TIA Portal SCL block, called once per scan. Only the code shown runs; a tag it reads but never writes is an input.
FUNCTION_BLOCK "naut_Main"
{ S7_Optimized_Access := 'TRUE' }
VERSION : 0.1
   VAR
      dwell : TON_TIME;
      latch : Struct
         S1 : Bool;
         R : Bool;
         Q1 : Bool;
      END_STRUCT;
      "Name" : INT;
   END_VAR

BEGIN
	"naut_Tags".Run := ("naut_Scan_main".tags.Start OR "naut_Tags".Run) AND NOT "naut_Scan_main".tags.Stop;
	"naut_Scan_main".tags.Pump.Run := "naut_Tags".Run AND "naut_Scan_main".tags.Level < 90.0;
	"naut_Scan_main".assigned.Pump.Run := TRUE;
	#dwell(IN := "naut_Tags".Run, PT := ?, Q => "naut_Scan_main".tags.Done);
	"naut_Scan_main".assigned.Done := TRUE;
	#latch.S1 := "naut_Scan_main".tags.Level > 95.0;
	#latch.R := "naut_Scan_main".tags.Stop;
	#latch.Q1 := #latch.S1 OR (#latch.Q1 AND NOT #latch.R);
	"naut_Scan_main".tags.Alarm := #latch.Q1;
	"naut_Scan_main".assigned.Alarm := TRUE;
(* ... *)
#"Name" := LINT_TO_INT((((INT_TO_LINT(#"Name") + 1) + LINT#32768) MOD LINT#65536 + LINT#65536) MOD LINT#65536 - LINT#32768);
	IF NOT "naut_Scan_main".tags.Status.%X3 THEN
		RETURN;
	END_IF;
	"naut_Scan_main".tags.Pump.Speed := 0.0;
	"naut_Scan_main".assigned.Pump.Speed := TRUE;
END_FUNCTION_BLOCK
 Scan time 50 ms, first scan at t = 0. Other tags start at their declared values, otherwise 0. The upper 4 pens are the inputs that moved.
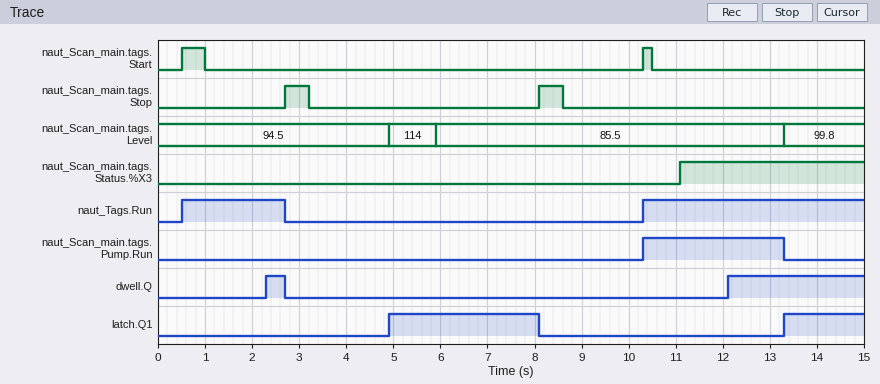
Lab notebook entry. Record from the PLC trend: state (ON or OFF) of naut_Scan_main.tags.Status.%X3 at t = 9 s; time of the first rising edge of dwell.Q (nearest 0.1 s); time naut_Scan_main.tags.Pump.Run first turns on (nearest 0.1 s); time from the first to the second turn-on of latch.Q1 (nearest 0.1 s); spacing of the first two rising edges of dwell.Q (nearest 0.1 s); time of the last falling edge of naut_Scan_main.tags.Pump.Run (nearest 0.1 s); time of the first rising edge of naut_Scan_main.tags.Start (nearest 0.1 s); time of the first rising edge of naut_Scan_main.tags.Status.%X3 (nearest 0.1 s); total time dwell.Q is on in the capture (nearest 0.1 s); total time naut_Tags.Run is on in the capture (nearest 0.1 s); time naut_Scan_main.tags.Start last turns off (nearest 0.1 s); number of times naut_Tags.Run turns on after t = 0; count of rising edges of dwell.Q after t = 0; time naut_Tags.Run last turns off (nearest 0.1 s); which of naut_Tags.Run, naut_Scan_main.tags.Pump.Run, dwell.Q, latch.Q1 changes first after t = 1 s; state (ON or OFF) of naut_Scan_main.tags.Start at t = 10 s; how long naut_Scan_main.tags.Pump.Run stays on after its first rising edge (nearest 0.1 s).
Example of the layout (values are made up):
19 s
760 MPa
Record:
OFF
2.3 s
10.3 s
8.4 s
9.8 s
13.3 s
0.5 s
11.1 s
3.3 s
6.9 s
10.5 s
2
2
2.7 s
dwell.Q
OFF
3.0 s
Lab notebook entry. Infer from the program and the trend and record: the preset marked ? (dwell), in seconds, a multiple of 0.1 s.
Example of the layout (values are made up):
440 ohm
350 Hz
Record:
1.8 s
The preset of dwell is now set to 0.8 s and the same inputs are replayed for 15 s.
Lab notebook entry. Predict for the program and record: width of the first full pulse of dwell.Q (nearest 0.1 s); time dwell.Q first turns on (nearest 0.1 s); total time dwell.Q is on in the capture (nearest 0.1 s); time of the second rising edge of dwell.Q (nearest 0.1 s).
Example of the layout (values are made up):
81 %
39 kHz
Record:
1.4 s
1.3 s
5.3 s
11.1 s
